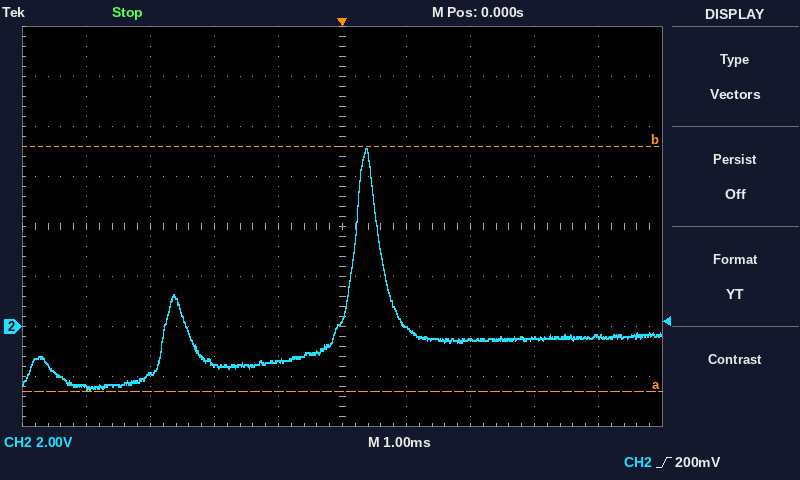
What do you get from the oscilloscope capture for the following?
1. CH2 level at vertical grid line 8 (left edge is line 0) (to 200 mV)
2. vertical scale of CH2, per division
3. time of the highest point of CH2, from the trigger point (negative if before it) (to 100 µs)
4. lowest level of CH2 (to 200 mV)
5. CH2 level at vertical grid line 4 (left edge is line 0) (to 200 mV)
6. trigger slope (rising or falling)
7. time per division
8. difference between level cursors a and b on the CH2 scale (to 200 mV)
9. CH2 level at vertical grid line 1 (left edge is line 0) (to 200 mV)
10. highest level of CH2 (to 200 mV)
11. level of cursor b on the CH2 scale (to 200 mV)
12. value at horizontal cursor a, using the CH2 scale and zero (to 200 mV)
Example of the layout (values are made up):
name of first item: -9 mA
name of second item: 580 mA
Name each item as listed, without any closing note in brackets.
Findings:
CH2 level at vertical grid line 8 (left edge is line 0): -400 mV
vertical scale of CH2, per division: 2 V
time of the highest point of CH2, from the trigger point (negative if before it): +400 µs
lowest level of CH2: -2.6 V
CH2 level at vertical grid line 4 (left edge is line 0): -1.4 V
trigger slope: rising
time per division: 1 ms
difference between level cursors a and b on the CH2 scale: 9.8 V
CH2 level at vertical grid line 1 (left edge is line 0): -2.4 V
highest level of CH2: 7.2 V
level of cursor b on the CH2 scale: 7.2 V
value at horizontal cursor a, using the CH2 scale and zero: -2.6 V
